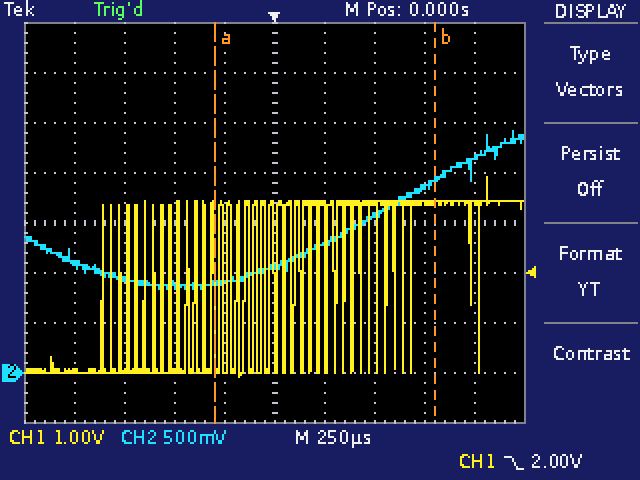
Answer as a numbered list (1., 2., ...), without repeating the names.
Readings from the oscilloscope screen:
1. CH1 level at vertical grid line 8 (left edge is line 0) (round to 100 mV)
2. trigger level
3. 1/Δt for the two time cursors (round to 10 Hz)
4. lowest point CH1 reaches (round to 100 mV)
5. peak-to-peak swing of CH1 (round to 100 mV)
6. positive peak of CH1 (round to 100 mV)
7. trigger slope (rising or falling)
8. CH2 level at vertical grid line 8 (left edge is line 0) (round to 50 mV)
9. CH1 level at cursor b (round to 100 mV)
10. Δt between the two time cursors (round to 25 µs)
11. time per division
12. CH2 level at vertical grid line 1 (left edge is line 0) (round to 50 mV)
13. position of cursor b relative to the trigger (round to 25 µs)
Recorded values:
1. 3.4 V
2. 2.00 V
3. 910 Hz
4. -100 mV
5. 4.0 V
6. 3.9 V
7. falling
8. 1.85 V
9. 3.4 V
10. 1.100 ms
11. 250 µs
12. 1.10 V
13. +800 µs
